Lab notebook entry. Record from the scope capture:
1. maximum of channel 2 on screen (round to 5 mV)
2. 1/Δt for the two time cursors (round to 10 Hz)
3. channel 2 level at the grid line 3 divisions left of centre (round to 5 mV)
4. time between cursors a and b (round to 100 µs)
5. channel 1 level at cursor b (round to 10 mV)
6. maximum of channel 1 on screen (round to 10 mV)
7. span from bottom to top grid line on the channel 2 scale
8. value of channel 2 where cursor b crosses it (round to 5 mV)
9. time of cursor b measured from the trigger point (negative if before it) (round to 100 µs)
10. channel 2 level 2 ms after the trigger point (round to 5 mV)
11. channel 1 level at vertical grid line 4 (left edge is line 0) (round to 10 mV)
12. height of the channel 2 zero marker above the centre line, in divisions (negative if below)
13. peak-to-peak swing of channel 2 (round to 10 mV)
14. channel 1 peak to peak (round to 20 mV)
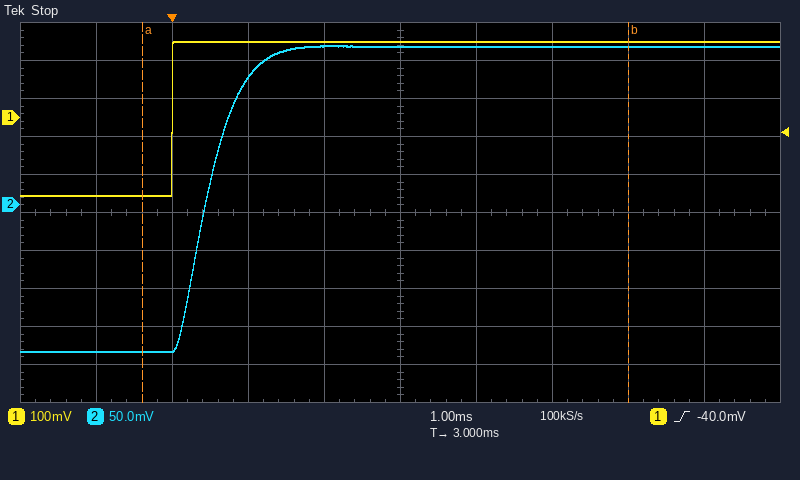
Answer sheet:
210 mV
160 Hz
-190 mV
6.4 ms
200 mV
200 mV
500 mV
210 mV
+6.0 ms
210 mV
200 mV
+0.2 div
400 mV
400 mV
